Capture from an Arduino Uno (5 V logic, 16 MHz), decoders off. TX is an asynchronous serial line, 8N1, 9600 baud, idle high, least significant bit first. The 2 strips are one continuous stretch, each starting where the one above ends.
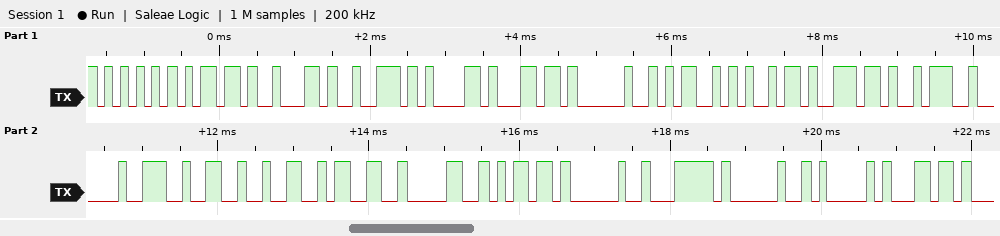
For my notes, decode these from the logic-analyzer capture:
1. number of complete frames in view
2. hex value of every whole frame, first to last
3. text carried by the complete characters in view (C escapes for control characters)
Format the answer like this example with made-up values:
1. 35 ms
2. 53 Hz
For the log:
1. 22
2. 55 6D 62 72 61 6C 20 4D 69 6E 3A 20 32 32 33 30 6D 20 7C 20 41 6C
3. "Umbral Min: 2230m | Al"
